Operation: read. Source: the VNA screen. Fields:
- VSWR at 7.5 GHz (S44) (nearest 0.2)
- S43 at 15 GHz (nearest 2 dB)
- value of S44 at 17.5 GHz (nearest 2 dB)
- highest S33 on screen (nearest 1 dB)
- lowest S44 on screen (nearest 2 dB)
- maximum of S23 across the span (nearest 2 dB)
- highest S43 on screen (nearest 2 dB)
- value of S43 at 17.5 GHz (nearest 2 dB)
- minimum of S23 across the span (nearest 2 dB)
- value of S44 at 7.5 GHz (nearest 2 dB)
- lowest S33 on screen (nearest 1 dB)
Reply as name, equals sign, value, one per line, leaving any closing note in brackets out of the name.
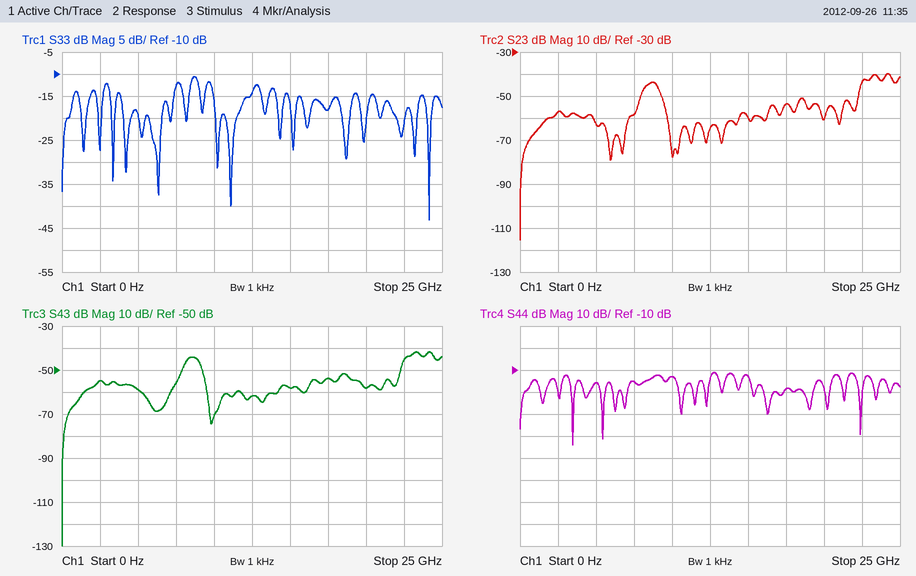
VSWR at 7.5 GHz (S44) = 1.4
S43 at 15 GHz = -58 dB
value of S44 at 17.5 GHz = -18 dB
highest S33 on screen = -11 dB
lowest S44 on screen = -44 dB
maximum of S23 across the span = -40 dB
highest S43 on screen = -42 dB
value of S43 at 17.5 GHz = -54 dB
minimum of S23 across the span = -116 dB
value of S44 at 7.5 GHz = -16 dB
lowest S33 on screen = -43 dB
